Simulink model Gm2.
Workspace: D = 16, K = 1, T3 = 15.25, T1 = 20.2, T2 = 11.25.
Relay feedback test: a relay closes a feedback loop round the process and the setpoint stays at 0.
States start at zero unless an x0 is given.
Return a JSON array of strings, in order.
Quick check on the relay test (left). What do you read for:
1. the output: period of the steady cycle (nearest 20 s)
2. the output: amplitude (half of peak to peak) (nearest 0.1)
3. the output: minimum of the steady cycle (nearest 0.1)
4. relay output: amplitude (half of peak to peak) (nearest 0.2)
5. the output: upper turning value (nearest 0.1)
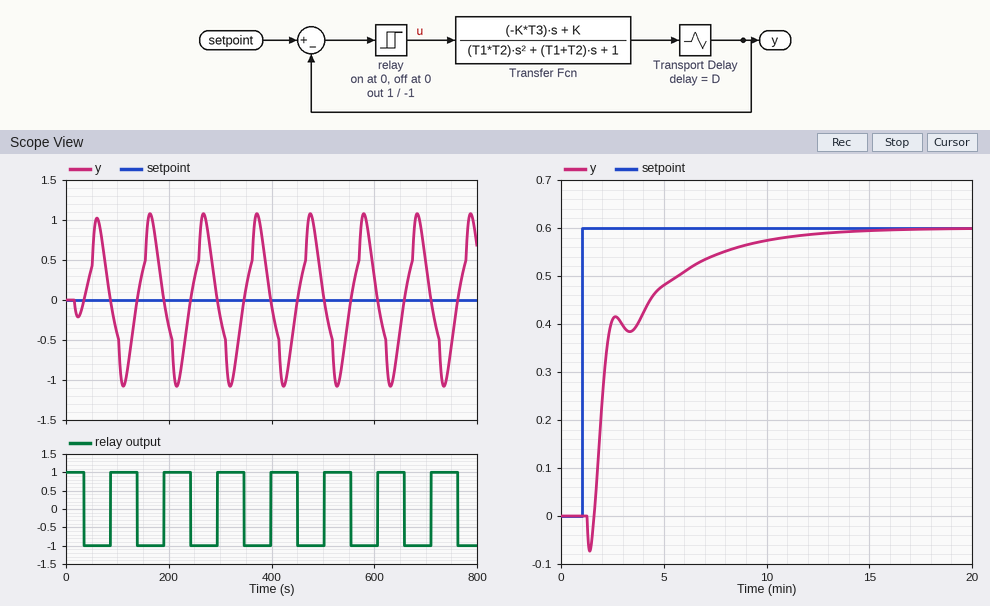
["100 s", "1.1", "-1.1", "1.0", "1.1"]
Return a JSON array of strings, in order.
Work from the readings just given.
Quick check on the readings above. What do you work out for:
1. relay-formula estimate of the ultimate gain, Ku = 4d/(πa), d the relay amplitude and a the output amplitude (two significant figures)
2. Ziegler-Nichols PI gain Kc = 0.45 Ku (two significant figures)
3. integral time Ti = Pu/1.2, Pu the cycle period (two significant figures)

["1.2", "0.54", "83 s"]
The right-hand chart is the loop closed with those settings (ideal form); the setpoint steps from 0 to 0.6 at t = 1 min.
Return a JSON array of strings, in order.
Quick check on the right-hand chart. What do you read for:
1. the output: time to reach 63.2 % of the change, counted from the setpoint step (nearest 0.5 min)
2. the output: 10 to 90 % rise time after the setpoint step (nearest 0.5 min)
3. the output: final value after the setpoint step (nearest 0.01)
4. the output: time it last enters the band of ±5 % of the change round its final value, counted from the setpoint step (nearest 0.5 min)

["1.5 min", "5.5 min", "0.60", "8.5 min"]
